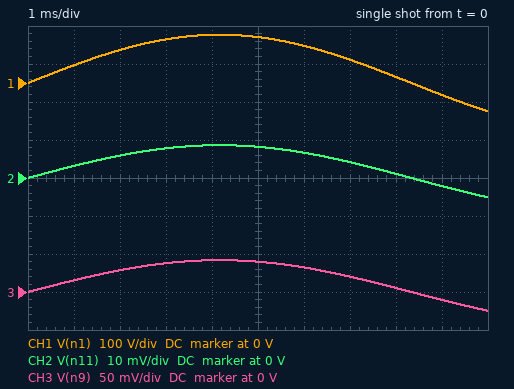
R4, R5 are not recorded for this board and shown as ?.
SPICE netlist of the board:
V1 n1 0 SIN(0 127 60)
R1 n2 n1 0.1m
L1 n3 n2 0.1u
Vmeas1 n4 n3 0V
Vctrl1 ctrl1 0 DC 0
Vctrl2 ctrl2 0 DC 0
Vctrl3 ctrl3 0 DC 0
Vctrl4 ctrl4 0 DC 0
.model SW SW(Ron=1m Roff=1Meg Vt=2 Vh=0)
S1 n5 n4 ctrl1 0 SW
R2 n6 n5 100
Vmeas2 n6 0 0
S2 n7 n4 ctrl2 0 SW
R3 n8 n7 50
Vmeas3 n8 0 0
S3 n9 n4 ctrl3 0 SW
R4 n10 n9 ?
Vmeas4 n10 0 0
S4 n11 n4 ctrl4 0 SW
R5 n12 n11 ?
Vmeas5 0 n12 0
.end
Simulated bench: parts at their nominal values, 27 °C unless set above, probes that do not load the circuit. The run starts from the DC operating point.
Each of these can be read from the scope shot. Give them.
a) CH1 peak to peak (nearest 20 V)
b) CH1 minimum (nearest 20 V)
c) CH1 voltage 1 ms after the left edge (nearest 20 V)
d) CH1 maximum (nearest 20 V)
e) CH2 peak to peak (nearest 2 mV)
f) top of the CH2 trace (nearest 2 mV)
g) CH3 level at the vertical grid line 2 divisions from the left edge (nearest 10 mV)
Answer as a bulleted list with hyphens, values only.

- 200 V
- -80 V
- 40 V
- 120 V
- 14 mV
- 8 mV
- 30 mV
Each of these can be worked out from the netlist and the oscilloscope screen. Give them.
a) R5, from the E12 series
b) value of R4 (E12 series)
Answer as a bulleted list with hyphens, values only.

- 68 Ω
- 330 Ω
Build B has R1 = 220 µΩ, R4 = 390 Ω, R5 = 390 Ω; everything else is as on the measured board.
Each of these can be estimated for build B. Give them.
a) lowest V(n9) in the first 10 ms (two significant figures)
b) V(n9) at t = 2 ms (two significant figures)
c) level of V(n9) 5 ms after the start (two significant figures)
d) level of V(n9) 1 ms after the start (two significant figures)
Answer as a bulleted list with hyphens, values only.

- -29 mV
- 34 mV
- 47 mV
- 18 mV
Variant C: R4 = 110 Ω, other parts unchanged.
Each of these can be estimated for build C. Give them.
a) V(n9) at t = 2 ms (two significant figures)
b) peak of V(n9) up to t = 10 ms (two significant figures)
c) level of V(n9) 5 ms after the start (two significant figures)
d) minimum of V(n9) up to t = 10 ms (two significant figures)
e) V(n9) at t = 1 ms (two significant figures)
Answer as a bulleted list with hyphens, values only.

- 9.6 mV
- 14 mV
- 13 mV
- -8.2 mV
- 5.1 mV
